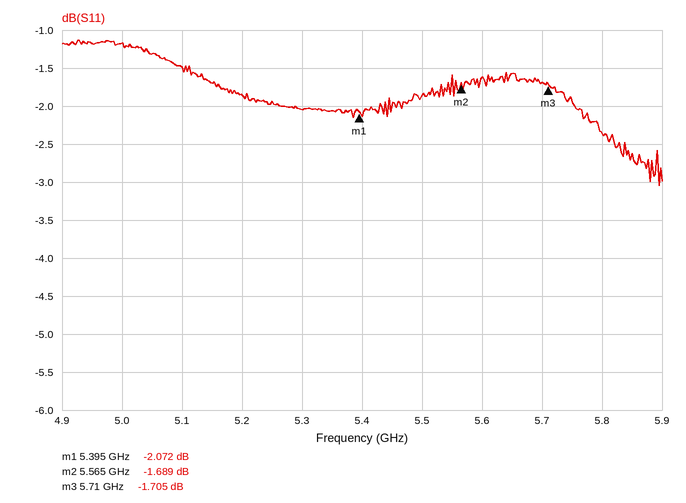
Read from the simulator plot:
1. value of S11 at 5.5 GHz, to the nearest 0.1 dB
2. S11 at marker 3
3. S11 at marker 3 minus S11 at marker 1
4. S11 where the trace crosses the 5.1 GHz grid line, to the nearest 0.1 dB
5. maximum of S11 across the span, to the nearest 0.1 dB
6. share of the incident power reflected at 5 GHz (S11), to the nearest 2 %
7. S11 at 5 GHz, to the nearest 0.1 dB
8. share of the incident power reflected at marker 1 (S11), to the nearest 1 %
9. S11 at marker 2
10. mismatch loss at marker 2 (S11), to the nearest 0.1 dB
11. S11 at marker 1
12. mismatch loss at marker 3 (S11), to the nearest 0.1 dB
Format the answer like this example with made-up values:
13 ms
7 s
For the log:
-1.9 dB
-1.705 dB
0.367 dB
-1.5 dB
-1.1 dB
76 %
-1.2 dB
62 %
-1.689 dB
4.9 dB
-2.072 dB
4.9 dB
